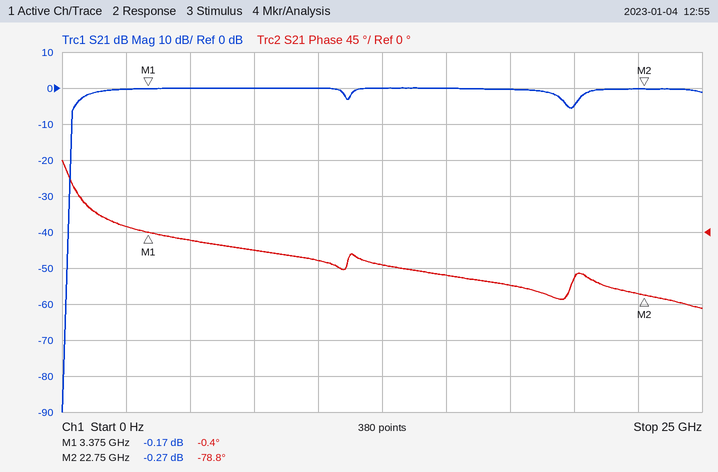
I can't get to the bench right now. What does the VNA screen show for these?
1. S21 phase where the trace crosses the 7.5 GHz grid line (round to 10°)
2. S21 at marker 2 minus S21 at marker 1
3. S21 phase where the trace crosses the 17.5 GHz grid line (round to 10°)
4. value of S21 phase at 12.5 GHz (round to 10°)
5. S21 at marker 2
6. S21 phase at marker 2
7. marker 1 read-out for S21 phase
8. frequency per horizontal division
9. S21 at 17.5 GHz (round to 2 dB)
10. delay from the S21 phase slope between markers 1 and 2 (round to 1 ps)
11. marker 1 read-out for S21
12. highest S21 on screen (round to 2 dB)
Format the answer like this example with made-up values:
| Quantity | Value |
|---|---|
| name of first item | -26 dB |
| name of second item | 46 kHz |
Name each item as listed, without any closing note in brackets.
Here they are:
| Quantity | Value |
|---|---|
| S21 phase where the trace crosses the 7.5 GHz grid line | -20° |
| S21 at marker 2 minus S21 at marker 1 | -0.10 dB |
| S21 phase where the trace crosses the 17.5 GHz grid line | -70° |
| value of S21 phase at 12.5 GHz | -40° |
| S21 at marker 2 | -0.27 dB |
| S21 phase at marker 2 | -78.8° |
| marker 1 read-out for S21 phase | -0.4° |
| frequency per horizontal division | 2.5 GHz |
| S21 at 17.5 GHz | 0 dB |
| delay from the S21 phase slope between markers 1 and 2 | 11 ps |
| marker 1 read-out for S21 | -0.17 dB |
| highest S21 on screen | 0 dB |
